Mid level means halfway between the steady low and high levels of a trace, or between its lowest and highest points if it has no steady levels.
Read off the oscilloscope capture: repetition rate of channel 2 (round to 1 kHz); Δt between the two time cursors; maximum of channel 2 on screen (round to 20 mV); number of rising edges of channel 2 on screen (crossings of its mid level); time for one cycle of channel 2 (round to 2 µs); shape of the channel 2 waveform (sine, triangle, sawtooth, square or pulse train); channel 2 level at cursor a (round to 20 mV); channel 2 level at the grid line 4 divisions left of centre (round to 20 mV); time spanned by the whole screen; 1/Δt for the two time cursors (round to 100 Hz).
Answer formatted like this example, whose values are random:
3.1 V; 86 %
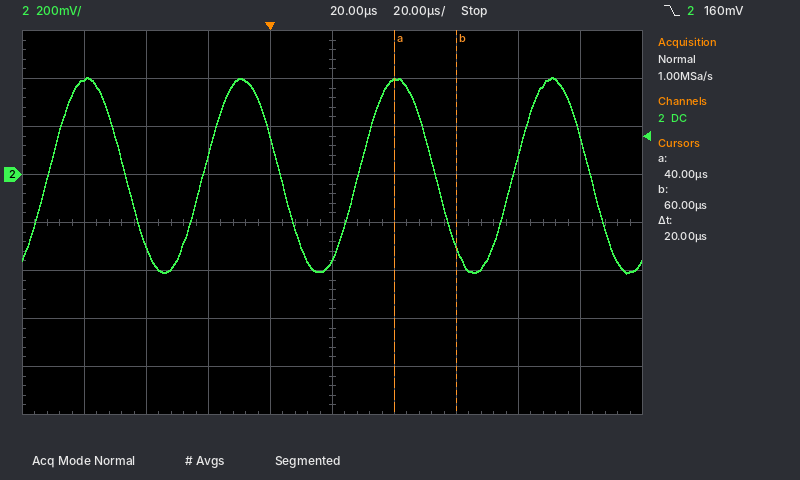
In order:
20 kHz; 20 µs; 400 mV; 4; 50 µs; sine; 400 mV; 400 mV; 200 µs; 50.0 kHz
